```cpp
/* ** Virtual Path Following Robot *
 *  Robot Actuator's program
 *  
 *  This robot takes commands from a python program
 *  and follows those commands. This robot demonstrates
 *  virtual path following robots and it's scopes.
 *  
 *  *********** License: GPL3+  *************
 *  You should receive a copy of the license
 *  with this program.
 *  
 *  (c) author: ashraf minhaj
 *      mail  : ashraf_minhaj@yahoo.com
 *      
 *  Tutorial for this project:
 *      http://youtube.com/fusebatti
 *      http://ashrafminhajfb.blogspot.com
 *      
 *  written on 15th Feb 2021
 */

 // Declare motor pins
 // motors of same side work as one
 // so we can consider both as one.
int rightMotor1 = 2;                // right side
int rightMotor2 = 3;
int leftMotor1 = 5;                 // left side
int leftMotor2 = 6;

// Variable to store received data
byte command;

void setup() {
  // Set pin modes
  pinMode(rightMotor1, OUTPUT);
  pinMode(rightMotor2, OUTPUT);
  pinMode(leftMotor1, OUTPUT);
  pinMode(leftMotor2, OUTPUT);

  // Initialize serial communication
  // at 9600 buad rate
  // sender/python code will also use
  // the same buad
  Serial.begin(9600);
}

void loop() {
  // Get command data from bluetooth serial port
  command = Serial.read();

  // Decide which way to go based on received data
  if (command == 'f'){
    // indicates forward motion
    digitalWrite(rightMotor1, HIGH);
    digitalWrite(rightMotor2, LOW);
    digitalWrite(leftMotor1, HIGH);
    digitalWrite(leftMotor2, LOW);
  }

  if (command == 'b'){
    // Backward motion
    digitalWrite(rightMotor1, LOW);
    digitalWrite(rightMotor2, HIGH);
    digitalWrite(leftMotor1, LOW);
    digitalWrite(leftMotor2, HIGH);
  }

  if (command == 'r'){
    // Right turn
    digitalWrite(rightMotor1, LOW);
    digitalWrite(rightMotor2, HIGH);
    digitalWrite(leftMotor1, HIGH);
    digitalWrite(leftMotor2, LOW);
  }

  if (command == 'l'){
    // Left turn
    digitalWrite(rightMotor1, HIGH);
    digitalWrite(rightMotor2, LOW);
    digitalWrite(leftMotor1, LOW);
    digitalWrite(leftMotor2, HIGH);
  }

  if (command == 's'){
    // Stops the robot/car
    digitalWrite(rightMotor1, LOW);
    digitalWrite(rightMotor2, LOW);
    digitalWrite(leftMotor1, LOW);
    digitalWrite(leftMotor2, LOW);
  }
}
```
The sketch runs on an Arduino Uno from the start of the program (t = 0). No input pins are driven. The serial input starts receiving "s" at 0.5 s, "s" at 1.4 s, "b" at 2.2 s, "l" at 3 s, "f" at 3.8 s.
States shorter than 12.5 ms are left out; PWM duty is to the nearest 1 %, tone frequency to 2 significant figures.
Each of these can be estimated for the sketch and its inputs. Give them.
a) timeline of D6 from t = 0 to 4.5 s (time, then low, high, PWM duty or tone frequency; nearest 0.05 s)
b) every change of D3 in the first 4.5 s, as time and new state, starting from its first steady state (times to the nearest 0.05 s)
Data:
0 s low; 2.2 s high; 3.8 s low
0 s low; 2.2 s high; 3 s low
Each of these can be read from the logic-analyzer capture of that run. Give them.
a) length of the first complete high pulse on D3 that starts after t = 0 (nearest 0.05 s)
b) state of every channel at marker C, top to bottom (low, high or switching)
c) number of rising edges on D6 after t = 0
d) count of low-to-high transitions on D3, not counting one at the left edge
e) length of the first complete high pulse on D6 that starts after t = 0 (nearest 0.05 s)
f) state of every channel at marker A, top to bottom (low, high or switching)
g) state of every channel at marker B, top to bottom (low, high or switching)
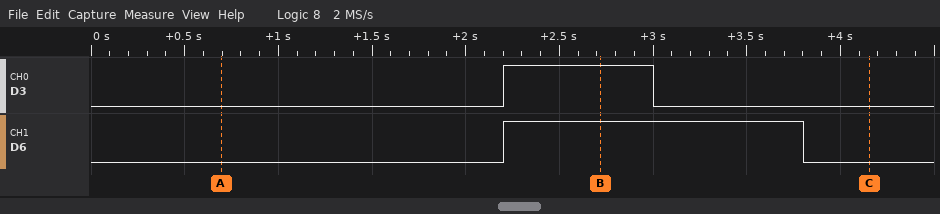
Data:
0.80 s
D3 low, D6 low
1
1
1.60 s
D3 low, D6 low
D3 high, D6 high
